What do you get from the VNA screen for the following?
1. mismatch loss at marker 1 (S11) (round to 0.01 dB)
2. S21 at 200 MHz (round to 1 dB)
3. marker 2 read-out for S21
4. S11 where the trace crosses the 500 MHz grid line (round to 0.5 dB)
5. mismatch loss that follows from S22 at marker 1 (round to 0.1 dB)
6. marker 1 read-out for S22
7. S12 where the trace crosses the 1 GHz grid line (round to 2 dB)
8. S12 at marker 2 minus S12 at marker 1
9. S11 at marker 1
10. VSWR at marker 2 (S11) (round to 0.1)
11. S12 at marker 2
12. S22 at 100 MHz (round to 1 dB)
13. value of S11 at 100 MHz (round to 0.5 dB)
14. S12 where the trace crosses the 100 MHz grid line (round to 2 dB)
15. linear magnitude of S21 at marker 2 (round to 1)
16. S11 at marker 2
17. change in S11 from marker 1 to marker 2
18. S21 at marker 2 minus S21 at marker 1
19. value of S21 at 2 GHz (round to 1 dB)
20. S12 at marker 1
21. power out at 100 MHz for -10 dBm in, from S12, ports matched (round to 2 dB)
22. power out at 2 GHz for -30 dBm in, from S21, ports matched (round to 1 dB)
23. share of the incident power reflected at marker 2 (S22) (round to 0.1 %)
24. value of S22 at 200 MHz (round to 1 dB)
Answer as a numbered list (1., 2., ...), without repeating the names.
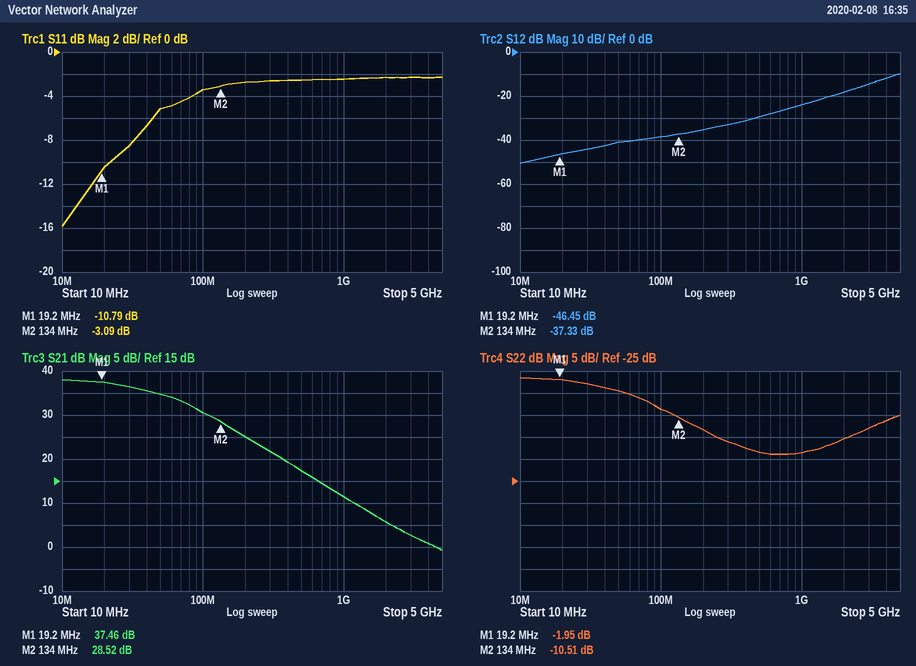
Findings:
1. 0.38 dB
2. 25 dB
3. 28.52 dB
4. -2.5 dB
5. 4.4 dB
6. -1.95 dB
7. -24 dB
8. 9.12 dB
9. -10.79 dB
10. 5.7
11. -37.33 dB
12. -9 dB
13. -3.5 dB
14. -38 dB
15. 27
16. -3.09 dB
17. 7.70 dB
18. -8.94 dB
19. 6 dB
20. -46.45 dB
21. -48 dBm
22. -24 dBm
23. 8.9 %
24. -13 dB
